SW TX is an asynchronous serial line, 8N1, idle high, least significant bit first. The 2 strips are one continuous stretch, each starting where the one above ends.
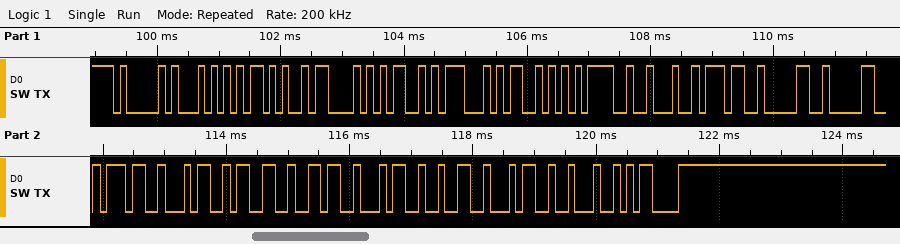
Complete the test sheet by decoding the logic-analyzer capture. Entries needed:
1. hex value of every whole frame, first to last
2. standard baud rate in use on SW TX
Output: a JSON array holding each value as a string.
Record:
["41 54 2B 43 4D 47 53 3D 22 37 30 30 37 34 33 36 34 32 34 22 0D", "9600 baud"]
